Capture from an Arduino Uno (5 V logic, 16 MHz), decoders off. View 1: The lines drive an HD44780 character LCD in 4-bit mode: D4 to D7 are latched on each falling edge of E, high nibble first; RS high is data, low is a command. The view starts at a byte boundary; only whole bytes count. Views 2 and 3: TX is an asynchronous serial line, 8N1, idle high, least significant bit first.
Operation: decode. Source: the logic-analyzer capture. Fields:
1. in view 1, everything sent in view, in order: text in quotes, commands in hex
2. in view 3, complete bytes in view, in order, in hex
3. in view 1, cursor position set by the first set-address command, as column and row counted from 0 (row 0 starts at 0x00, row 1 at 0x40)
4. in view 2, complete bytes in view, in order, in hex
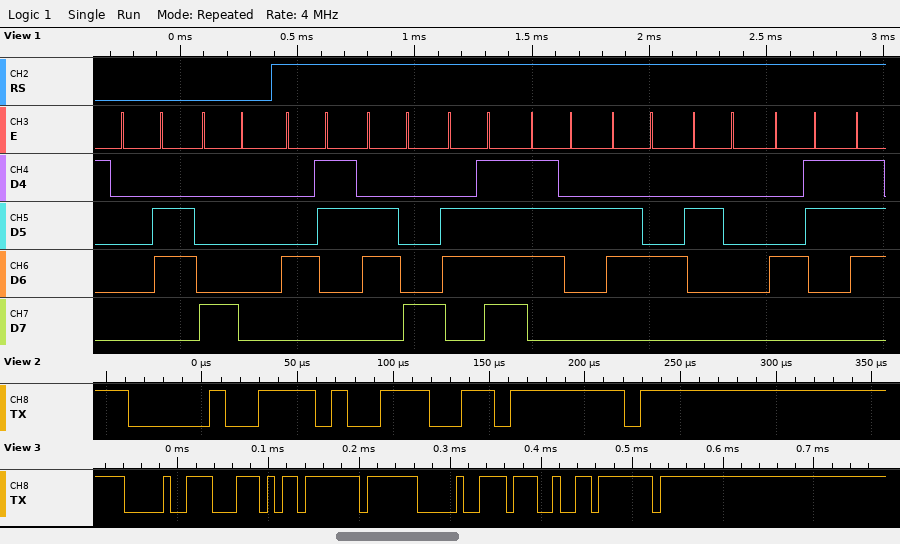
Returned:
0x06 0x80 "Chord C"
0x90 0x5C 0x7F 0x90 0x27 0x7F
column 0, row 0
90 39 7F
